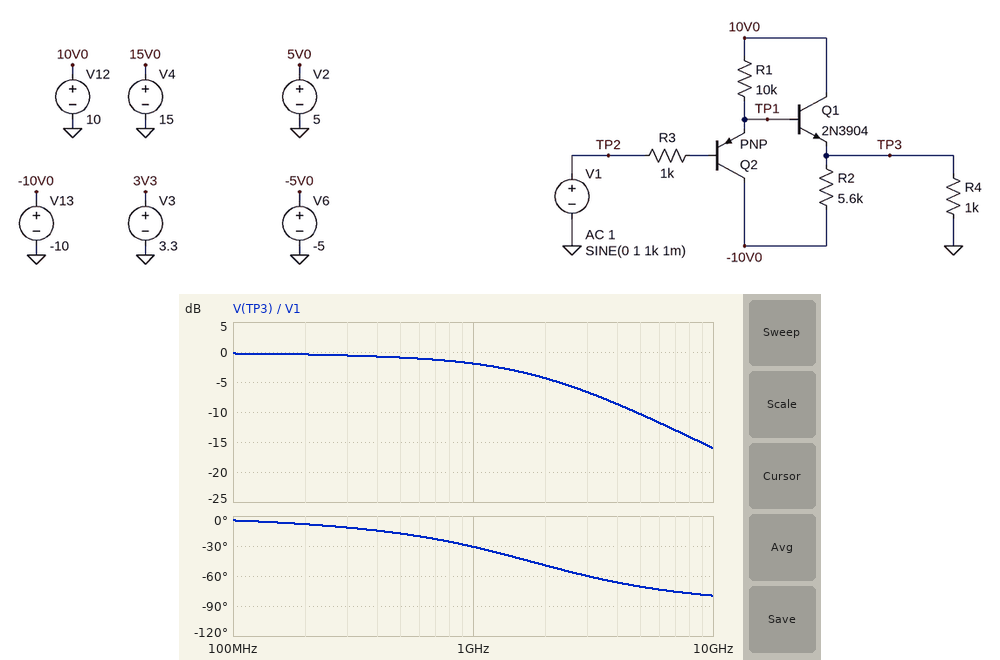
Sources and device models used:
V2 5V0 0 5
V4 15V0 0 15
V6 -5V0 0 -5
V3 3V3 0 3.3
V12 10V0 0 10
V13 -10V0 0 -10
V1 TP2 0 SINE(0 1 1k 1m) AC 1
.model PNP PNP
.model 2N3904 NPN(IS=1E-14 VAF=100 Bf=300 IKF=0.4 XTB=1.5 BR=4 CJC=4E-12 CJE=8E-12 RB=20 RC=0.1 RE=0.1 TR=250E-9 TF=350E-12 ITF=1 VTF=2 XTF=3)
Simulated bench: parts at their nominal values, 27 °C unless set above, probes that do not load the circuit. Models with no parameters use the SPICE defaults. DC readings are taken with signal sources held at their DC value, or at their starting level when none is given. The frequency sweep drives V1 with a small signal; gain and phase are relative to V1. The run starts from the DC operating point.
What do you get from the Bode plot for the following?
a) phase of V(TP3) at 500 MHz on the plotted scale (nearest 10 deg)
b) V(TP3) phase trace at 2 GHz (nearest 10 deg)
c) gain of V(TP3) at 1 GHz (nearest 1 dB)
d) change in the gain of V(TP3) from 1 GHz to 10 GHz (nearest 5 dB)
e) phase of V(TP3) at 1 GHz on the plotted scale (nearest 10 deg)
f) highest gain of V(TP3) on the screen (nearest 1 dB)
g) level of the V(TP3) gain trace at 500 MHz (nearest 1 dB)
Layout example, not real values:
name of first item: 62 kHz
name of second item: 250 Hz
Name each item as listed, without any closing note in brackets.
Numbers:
phase of V(TP3) at 500 MHz on the plotted scale: -20 deg
V(TP3) phase trace at 2 GHz: -50 deg
gain of V(TP3) at 1 GHz: -2 dB
change in the gain of V(TP3) from 1 GHz to 10 GHz: -15 dB
phase of V(TP3) at 1 GHz on the plotted scale: -30 deg
highest gain of V(TP3) on the screen: 0 dB
level of the V(TP3) gain trace at 500 MHz: -1 dB
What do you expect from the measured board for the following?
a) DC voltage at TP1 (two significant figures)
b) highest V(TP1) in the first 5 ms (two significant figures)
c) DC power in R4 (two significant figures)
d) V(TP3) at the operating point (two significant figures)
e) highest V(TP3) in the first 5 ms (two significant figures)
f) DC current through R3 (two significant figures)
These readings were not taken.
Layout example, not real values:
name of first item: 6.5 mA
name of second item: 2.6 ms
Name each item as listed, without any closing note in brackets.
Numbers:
DC voltage at TP1: 780 mV
highest V(TP1) in the first 5 ms: 1.8 V
DC power in R4: 12 µW
V(TP3) at the operating point: 110 mV
highest V(TP3) in the first 5 ms: 1.1 V
DC current through R3: 9.1 µA
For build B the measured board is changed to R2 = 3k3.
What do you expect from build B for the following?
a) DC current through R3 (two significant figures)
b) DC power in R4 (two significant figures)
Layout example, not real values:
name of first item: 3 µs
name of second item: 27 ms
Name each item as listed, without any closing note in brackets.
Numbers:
DC current through R3: 9.0 µA
DC power in R4: 9.5 µW
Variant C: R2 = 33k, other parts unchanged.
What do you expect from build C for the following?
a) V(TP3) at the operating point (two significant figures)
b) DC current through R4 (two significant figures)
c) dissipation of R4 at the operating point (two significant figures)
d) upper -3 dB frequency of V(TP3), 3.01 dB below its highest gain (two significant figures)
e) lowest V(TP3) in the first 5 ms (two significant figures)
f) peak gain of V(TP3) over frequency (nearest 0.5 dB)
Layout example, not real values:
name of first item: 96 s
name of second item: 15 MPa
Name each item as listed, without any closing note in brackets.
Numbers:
V(TP3) at the operating point: 150 mV
DC current through R4: 150 µA
dissipation of R4 at the operating point: 22 µW
upper -3 dB frequency of V(TP3), 3.01 dB below its highest gain: 1.7 GHz
lowest V(TP3) in the first 5 ms: -290 mV
peak gain of V(TP3) over frequency: -0.5 dB
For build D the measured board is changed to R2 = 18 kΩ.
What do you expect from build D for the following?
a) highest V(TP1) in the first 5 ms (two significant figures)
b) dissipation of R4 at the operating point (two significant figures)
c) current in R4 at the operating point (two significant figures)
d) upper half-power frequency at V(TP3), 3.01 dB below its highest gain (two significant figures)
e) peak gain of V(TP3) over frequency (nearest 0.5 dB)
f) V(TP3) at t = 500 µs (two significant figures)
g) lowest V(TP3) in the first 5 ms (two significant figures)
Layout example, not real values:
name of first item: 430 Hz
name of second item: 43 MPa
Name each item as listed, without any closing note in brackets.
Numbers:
highest V(TP1) in the first 5 ms: 1.8 V
dissipation of R4 at the operating point: 19 µW
current in R4 at the operating point: 140 µA
upper half-power frequency at V(TP3), 3.01 dB below its highest gain: 1.6 GHz
peak gain of V(TP3) over frequency: -0.5 dB
V(TP3) at t = 500 µs: 140 mV
lowest V(TP3) in the first 5 ms: -530 mV
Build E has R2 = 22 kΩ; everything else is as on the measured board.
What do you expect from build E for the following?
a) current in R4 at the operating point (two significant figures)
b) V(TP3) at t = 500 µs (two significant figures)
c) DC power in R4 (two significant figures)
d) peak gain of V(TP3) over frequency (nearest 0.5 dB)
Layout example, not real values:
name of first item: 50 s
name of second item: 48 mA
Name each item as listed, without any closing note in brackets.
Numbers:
current in R4 at the operating point: 140 µA
V(TP3) at t = 500 µs: 140 mV
DC power in R4: 20 µW
peak gain of V(TP3) over frequency: -0.5 dB
